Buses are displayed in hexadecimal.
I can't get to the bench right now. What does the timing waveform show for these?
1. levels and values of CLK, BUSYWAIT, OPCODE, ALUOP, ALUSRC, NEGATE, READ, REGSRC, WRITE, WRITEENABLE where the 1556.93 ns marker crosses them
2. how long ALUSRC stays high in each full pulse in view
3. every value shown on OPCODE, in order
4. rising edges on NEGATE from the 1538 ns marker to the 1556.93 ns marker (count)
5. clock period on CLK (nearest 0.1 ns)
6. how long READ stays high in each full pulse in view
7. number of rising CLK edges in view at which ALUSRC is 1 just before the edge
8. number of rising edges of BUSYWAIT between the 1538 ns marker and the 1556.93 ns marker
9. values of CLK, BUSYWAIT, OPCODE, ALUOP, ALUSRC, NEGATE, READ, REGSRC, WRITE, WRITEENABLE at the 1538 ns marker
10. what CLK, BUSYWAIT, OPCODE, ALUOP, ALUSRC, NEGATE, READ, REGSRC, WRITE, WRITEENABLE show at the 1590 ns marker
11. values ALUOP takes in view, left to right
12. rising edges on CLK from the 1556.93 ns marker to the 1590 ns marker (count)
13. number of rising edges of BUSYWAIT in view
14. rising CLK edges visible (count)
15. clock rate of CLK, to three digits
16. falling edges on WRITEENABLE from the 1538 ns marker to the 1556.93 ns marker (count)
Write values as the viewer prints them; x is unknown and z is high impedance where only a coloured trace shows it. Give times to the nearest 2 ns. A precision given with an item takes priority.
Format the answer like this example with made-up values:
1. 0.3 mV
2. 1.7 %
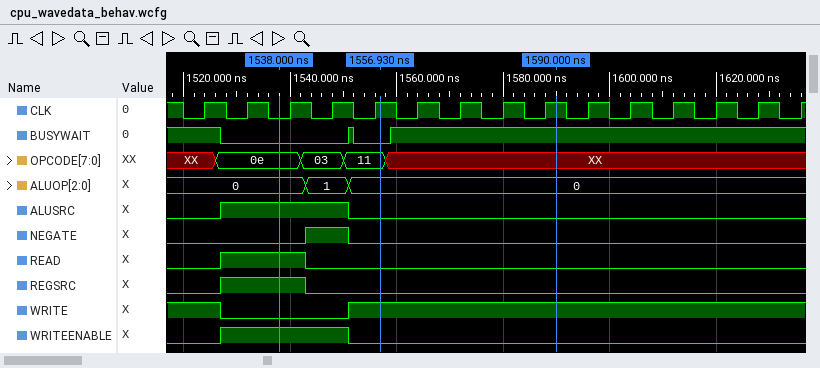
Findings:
1. CLK=1, BUSYWAIT=0, OPCODE=11, ALUOP=0, ALUSRC=0, NEGATE=0, READ=0, REGSRC=0, WRITE=1, WRITEENABLE=0
2. 24 ns
3. XX, 0e, 03, 11, XX
4. 1
5. 8 ns
6. 16 ns
7. 3
8. 1
9. CLK=0, BUSYWAIT=0, OPCODE=0e, ALUOP=0, ALUSRC=1, NEGATE=0, READ=1, REGSRC=1, WRITE=0, WRITEENABLE=1
10. CLK=1, BUSYWAIT=1, OPCODE=XX, ALUOP=0, ALUSRC=0, NEGATE=0, READ=0, REGSRC=0, WRITE=1, WRITEENABLE=0
11. 0, 1, 0
12. 4
13. 2
14. 15
15. 125 MHz
16. 1
